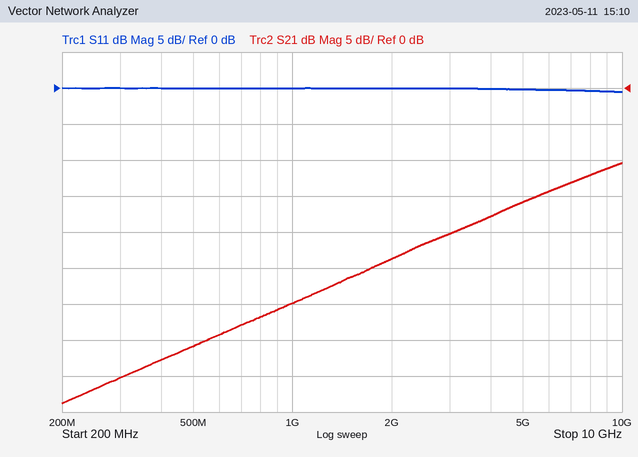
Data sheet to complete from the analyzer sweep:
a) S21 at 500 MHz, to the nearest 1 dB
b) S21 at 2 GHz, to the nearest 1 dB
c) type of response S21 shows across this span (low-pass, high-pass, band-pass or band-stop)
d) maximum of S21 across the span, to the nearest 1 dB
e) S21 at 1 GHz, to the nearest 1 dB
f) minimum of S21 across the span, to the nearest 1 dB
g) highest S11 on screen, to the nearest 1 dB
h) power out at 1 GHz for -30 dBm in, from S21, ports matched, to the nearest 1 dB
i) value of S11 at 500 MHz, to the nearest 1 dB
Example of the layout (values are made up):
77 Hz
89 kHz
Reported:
-36 dB
-24 dB
high-pass
-10 dB
-30 dB
-44 dB
0 dB
-60 dBm
0 dB
